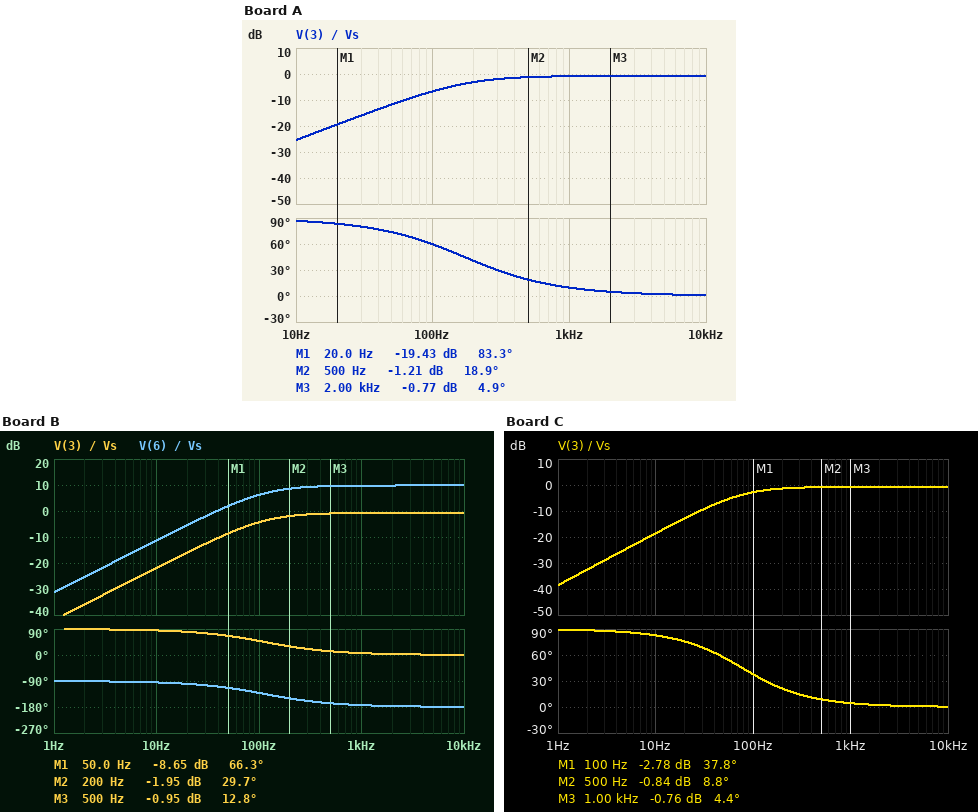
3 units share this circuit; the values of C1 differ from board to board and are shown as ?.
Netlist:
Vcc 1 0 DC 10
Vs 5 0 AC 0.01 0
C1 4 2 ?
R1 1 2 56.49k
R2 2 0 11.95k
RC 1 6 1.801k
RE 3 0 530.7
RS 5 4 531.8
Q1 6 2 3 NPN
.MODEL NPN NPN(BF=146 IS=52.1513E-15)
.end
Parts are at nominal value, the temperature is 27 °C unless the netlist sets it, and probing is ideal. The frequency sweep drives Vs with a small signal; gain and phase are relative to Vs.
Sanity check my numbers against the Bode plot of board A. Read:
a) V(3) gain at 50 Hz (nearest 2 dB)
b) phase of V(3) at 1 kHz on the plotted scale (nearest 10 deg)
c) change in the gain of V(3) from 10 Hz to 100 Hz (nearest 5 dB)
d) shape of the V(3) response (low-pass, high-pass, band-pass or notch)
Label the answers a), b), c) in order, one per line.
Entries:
a) -12 dB
b) 10 deg
c) 20 dB
d) high-pass
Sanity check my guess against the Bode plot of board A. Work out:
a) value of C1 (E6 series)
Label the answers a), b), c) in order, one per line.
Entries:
a) 100 nF
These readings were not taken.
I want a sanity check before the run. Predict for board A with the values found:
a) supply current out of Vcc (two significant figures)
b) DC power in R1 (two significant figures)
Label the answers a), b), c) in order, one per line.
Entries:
a) 2.0 mA
b) 1.2 mW
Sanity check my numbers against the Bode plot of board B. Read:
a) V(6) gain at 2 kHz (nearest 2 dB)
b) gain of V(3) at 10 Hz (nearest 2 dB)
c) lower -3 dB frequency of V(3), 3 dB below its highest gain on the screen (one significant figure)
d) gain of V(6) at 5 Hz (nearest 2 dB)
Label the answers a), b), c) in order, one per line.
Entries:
a) 10 dB
b) -22 dB
c) 100 Hz
d) -18 dB
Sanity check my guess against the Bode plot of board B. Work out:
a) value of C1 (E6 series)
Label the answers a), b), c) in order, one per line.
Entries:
a) 150 nF
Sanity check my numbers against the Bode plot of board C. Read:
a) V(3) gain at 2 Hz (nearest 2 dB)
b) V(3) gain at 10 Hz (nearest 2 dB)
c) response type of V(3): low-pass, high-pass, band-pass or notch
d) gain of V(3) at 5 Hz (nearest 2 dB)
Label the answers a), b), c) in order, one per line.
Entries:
a) -32 dB
b) -18 dB
c) high-pass
d) -24 dB
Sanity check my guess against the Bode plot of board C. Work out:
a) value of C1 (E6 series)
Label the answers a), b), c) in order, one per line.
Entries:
a) 220 nF
